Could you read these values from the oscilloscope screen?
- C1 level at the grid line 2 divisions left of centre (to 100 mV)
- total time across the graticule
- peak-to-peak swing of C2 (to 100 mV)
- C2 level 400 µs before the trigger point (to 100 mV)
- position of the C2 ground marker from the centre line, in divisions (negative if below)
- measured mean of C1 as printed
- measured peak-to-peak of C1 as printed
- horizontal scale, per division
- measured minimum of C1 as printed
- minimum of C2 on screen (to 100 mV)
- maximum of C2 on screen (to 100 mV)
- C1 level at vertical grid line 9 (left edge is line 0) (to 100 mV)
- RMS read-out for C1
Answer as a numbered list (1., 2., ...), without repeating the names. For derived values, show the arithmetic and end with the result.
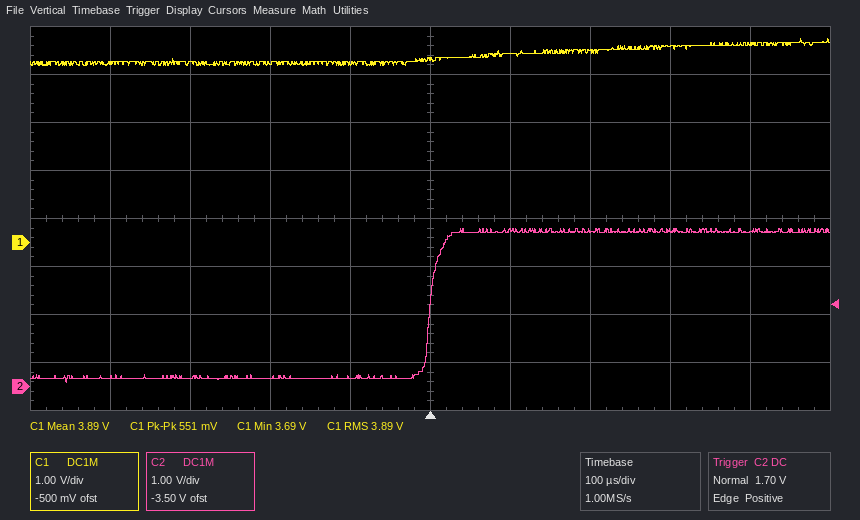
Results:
1. 3.7 V
2. 1 ms
3. 3.3 V − (100 mV) = 3.2 V
4. 200 mV
5. -3.5 div
6. 3.89 V
7. 551 mV
8. 100 µs
9. 3.69 V
10. 100 mV
11. 3.3 V
12. 4.1 V
13. 3.89 V
